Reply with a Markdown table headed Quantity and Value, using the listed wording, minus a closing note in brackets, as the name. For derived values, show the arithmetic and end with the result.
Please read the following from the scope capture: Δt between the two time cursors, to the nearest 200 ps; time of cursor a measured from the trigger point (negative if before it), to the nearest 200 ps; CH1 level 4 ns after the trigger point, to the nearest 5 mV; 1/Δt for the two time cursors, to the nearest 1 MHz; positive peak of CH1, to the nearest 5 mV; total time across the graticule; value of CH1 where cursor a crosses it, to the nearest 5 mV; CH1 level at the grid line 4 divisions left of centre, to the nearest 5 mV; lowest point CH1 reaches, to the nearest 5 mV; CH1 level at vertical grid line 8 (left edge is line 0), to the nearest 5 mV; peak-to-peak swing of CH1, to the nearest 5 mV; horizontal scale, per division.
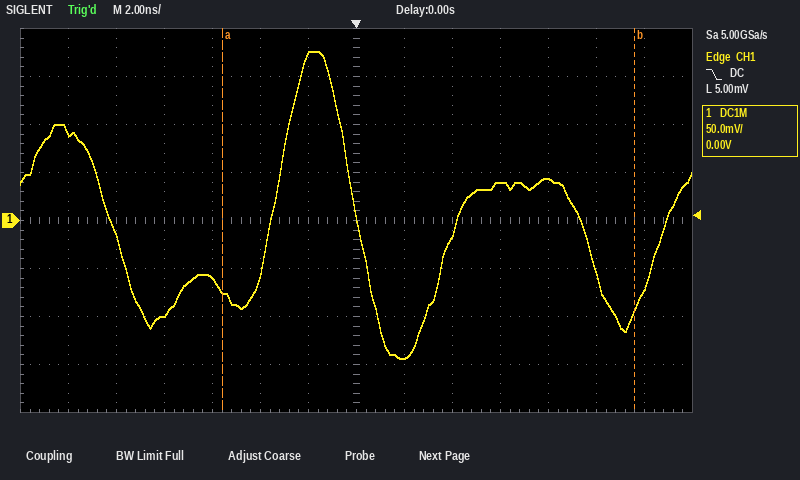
| Quantity | Value |
|---|---|
| Δt between the two time cursors, to the nearest 200 ps | 17.2 ns |
| time of cursor a measured from the trigger point (negative if before it), to the nearest 200 ps | -5.6 ns |
| CH1 level 4 ns after the trigger point, to the nearest 5 mV | -15 mV |
| 1/Δt for the two time cursors, to the nearest 1 MHz | 1 / 17.2 ns ≈ 58 MHz |
| positive peak of CH1, to the nearest 5 mV | 175 mV |
| total time across the graticule | 28 ns |
| value of CH1 where cursor a crosses it, to the nearest 5 mV | -75 mV |
| CH1 level at the grid line 4 divisions left of centre, to the nearest 5 mV | -100 mV |
| lowest point CH1 reaches, to the nearest 5 mV | -145 mV |
| CH1 level at vertical grid line 8 (left edge is line 0), to the nearest 5 mV | -145 mV |
| peak-to-peak swing of CH1, to the nearest 5 mV | 175 mV − (-145 mV) = 320 mV |
| horizontal scale, per division | 2 ns |
